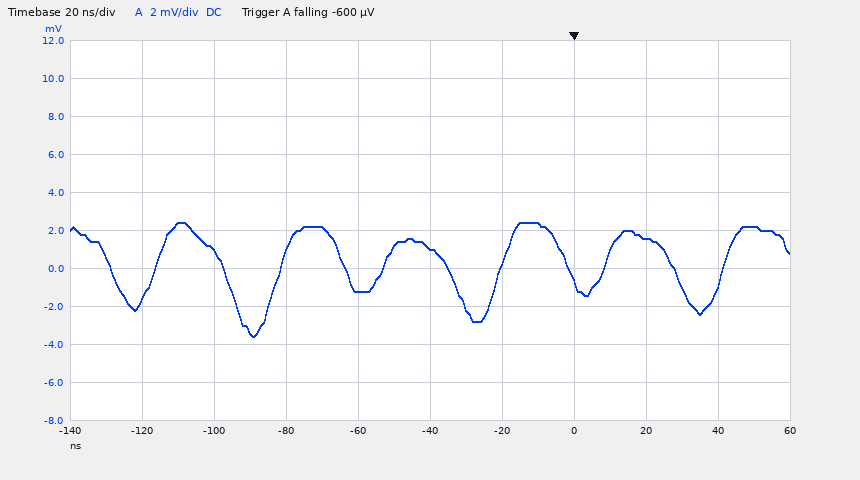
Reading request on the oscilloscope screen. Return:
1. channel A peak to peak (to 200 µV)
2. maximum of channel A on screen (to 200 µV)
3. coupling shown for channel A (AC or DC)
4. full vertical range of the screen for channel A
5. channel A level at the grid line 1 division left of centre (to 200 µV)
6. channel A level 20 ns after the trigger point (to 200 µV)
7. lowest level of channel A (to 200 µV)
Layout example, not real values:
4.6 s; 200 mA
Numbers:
6.0 mV; 2.4 mV; DC; 20 mV; -1.2 mV; 1.6 mV; -3.6 mV
